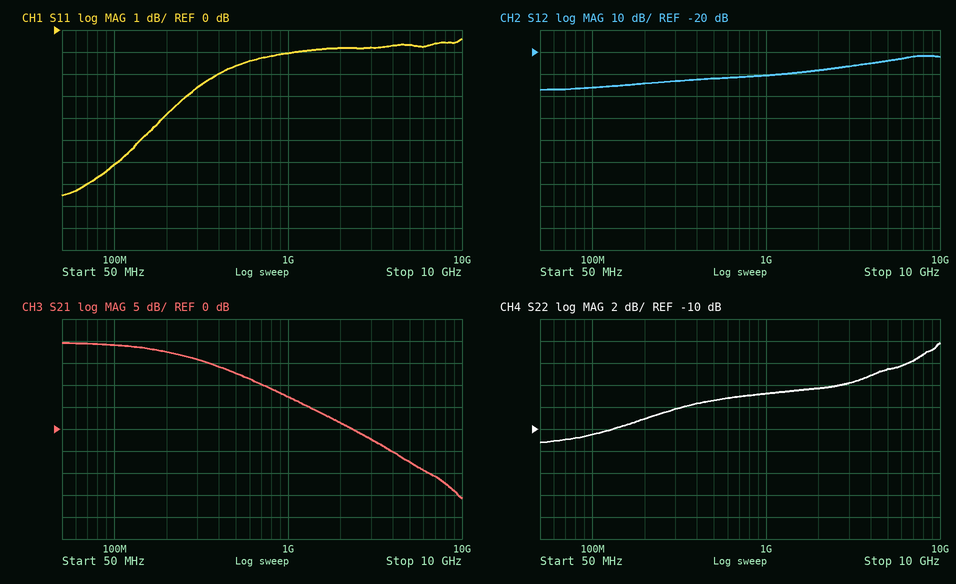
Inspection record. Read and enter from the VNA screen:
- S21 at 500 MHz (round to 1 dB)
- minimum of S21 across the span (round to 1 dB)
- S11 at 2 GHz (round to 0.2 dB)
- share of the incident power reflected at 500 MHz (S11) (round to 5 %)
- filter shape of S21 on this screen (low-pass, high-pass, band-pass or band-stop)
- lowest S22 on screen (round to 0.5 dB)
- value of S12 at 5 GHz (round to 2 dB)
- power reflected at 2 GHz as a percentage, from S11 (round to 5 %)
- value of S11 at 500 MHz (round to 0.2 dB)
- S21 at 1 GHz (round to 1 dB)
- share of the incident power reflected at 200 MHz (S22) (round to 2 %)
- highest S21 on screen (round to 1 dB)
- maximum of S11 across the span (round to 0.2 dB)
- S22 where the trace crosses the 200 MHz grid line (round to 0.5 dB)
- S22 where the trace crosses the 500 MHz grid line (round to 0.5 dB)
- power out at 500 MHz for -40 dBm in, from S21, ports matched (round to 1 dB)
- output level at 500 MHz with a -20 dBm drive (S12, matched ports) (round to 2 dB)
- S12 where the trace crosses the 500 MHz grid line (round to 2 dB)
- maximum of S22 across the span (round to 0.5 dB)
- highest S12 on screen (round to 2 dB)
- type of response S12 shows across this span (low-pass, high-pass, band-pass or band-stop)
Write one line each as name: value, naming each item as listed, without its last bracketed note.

S21 at 500 MHz: 13 dB
minimum of S21 across the span: -16 dB
S11 at 2 GHz: -0.8 dB
share of the incident power reflected at 500 MHz (S11): 70 %
filter shape of S21 on this screen: low-pass
lowest S22 on screen: -11.0 dB
value of S12 at 5 GHz: -24 dB
power reflected at 2 GHz as a percentage, from S11: 85 %
value of S11 at 500 MHz: -1.6 dB
S21 at 1 GHz: 7 dB
share of the incident power reflected at 200 MHz (S22): 12 %
highest S21 on screen: 20 dB
maximum of S11 across the span: -0.4 dB
S22 where the trace crosses the 200 MHz grid line: -9.0 dB
S22 where the trace crosses the 500 MHz grid line: -7.5 dB
power out at 500 MHz for -40 dBm in, from S21, ports matched: -27 dBm
output level at 500 MHz with a -20 dBm drive (S12, matched ports): -52 dBm
S12 where the trace crosses the 500 MHz grid line: -32 dB
maximum of S22 across the span: -2.0 dB
highest S12 on screen: -22 dB
type of response S12 shows across this span: high-pass
